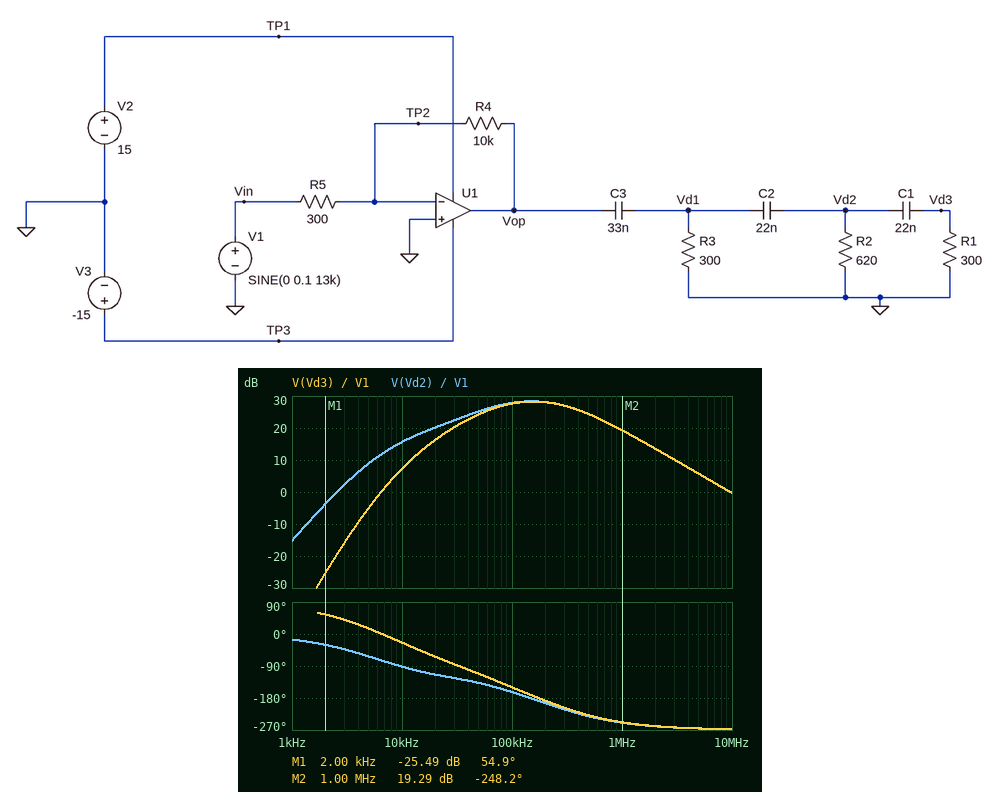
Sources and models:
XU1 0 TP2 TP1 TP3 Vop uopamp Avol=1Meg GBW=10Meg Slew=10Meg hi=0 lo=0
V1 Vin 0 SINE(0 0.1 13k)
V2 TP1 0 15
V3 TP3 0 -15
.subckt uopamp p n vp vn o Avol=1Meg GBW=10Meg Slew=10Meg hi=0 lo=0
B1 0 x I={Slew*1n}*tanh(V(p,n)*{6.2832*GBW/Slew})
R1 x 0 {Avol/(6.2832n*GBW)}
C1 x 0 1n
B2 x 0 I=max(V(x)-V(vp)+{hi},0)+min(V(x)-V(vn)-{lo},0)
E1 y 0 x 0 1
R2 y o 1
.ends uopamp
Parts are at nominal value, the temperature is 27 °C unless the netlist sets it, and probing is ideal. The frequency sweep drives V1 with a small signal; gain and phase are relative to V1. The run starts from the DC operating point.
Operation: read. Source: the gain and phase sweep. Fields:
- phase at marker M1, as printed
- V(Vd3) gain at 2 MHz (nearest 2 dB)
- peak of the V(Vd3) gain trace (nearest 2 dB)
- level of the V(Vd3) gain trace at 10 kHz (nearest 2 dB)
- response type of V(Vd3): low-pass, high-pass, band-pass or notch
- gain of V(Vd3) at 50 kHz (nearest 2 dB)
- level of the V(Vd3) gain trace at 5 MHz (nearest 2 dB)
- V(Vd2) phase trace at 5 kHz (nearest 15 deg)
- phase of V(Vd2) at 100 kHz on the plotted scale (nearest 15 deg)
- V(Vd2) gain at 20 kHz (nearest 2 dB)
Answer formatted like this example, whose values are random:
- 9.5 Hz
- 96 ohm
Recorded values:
- 54.9 deg
- 14 dB
- 28 dB
- 8 dB
- band-pass
- 24 dB
- 6 dB
- -60 deg
- -165 deg
- 20 dB
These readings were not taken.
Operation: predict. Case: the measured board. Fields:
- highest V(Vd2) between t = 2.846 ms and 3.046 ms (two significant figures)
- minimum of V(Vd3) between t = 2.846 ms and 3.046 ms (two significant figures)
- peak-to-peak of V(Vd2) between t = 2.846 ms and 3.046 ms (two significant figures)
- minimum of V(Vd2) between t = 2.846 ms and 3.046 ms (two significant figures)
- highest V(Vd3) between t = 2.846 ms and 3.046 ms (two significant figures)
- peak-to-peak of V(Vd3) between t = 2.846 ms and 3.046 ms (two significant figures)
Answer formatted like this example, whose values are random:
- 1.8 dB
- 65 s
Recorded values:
- 750 mV
- -360 mV
- 1.5 V
- -750 mV
- 360 mV
- 710 mV
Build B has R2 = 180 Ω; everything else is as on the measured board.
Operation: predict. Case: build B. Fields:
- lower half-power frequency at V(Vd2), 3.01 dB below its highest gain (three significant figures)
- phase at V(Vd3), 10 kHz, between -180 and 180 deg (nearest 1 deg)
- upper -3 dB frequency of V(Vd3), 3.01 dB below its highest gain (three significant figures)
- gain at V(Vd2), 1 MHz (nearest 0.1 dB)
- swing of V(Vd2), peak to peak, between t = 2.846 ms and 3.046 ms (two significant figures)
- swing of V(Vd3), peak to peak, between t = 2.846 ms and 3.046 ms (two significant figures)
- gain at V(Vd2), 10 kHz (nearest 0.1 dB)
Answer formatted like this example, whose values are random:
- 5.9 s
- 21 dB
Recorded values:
- 71.4 kHz
- 0 deg
- 486 kHz
- 19.2 dB
- 800 mV
- 380 mV
- 9.4 dB
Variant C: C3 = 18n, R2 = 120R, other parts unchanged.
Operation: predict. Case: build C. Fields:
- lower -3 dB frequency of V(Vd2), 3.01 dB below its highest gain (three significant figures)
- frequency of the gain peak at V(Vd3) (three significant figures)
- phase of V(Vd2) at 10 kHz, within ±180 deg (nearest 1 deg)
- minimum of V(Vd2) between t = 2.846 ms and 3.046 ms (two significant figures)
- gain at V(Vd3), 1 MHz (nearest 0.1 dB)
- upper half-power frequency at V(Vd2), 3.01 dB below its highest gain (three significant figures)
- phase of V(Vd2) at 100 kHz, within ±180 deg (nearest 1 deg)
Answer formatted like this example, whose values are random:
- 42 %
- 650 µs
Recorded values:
- 101 kHz
- 248 kHz
- -53 deg
- -190 mV
- 19.1 dB
- 597 kHz
- -131 deg
